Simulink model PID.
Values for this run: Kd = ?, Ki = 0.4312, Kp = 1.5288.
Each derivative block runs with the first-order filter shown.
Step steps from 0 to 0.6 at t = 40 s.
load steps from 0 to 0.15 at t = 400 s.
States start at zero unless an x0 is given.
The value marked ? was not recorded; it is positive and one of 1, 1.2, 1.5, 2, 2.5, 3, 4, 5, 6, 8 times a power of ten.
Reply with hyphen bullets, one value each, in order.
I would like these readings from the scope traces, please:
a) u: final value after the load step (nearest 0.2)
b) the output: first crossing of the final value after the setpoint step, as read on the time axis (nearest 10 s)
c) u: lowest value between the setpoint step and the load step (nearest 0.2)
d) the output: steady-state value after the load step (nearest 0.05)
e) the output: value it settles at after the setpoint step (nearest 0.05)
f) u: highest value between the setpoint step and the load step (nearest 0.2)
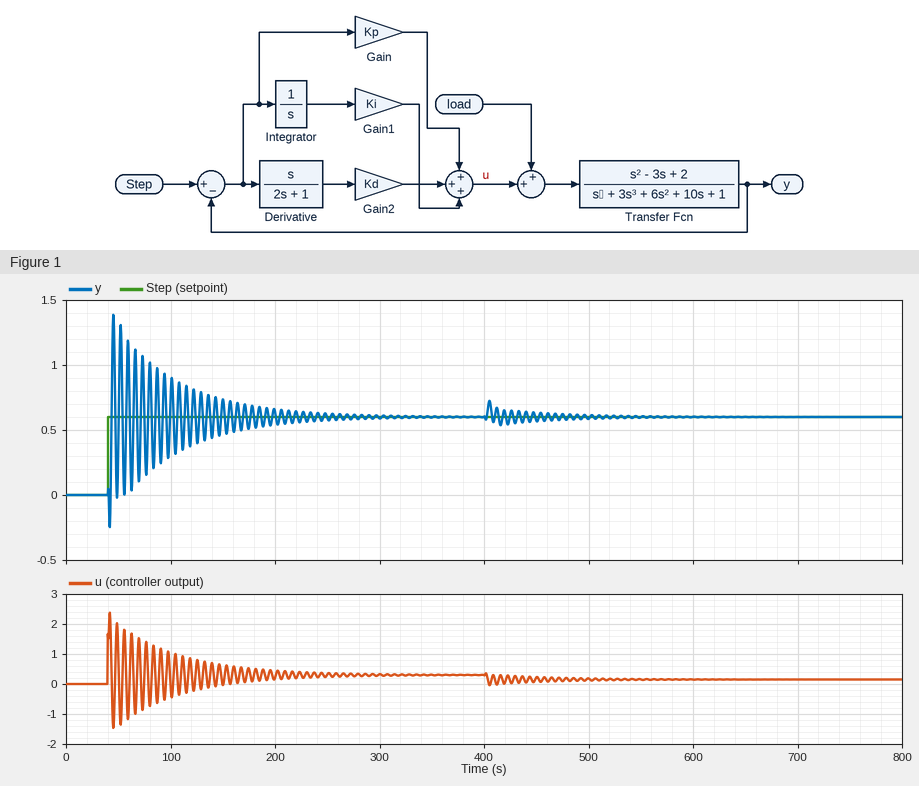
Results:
- 0.2
- 40 s
- -1.4
- 0.60
- 0.60
- 2.4
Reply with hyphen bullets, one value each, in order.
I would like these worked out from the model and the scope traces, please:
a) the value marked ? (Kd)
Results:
- 2.5
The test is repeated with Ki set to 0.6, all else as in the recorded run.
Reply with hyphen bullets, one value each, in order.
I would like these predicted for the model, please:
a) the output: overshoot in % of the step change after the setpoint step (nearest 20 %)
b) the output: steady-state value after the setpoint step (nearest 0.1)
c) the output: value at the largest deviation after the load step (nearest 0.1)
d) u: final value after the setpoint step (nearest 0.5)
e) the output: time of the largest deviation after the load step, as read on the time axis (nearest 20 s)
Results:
- 160 %
- 0.6
- 0.7
- 0.5
- 400 s
